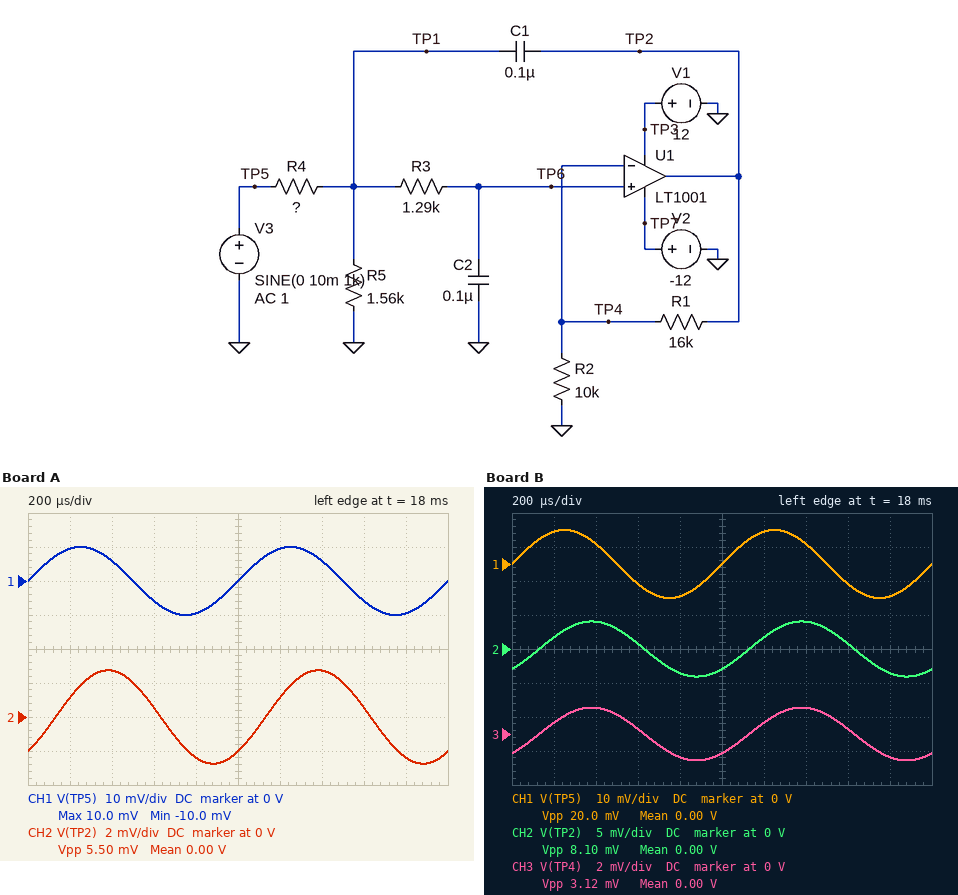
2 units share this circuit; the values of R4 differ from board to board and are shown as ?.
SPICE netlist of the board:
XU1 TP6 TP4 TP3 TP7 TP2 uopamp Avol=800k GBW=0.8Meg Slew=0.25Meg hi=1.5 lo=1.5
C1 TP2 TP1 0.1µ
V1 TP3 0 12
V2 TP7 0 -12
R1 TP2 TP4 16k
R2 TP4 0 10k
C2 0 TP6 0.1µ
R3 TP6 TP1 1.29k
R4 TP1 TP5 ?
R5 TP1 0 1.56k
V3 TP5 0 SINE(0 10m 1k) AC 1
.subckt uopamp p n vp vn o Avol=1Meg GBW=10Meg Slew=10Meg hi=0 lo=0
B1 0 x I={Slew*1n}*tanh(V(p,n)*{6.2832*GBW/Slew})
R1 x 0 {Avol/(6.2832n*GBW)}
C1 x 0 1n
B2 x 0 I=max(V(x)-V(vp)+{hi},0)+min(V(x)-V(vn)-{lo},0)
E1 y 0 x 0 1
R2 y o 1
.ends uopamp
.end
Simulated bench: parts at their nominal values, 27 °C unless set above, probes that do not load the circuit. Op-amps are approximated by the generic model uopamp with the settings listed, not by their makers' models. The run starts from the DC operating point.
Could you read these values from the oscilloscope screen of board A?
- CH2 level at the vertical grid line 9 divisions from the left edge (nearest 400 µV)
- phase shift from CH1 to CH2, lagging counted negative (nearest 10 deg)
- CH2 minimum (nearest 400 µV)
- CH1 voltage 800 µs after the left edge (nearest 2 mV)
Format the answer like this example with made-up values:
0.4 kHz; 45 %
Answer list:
-2.4 mV; -50 deg; -2.8 mV; -10 mV
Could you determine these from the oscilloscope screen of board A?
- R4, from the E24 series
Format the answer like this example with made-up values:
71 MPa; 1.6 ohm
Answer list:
43 kΩ
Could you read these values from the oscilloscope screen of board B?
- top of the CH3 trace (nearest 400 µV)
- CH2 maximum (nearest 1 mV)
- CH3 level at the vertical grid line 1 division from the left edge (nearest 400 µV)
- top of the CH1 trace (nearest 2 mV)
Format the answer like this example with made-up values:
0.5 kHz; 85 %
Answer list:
1.6 mV; 4 mV; 800 µV; 10 mV
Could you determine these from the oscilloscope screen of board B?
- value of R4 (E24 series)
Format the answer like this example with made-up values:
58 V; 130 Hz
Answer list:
27 kΩ
